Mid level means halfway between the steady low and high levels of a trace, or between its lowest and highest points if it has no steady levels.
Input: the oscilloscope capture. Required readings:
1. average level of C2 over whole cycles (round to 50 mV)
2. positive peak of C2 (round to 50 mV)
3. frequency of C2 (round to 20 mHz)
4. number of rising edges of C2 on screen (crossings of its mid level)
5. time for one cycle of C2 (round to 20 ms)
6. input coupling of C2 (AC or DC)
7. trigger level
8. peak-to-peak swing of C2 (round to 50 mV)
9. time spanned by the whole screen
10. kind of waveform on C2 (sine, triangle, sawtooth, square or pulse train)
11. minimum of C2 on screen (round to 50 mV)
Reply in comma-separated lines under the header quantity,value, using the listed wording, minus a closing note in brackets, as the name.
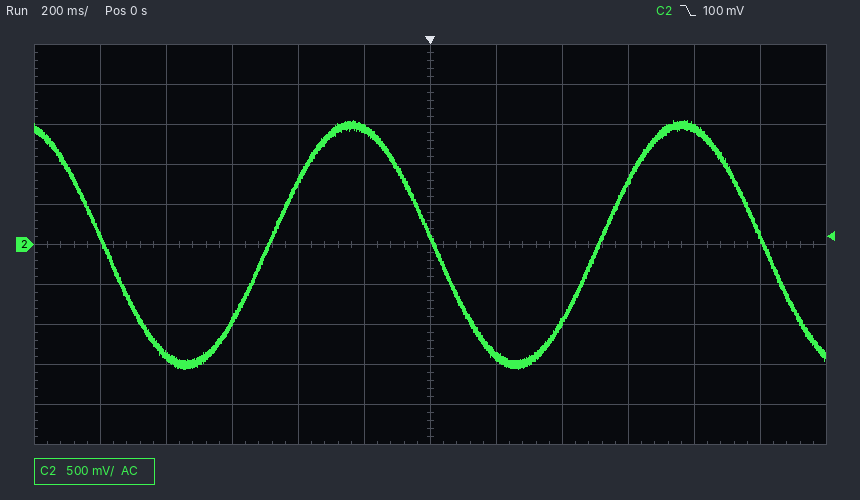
quantity,value
average level of C2 over whole cycles,0 mV
positive peak of C2,1.55 V
frequency of C2,1.00 Hz
number of rising edges of C2 on screen,2
time for one cycle of C2,1.00 s
input coupling of C2,AC
trigger level,100 mV
peak-to-peak swing of C2,3.10 V
time spanned by the whole screen,2.4 s
kind of waveform on C2,sine
minimum of C2 on screen,-1.55 V
